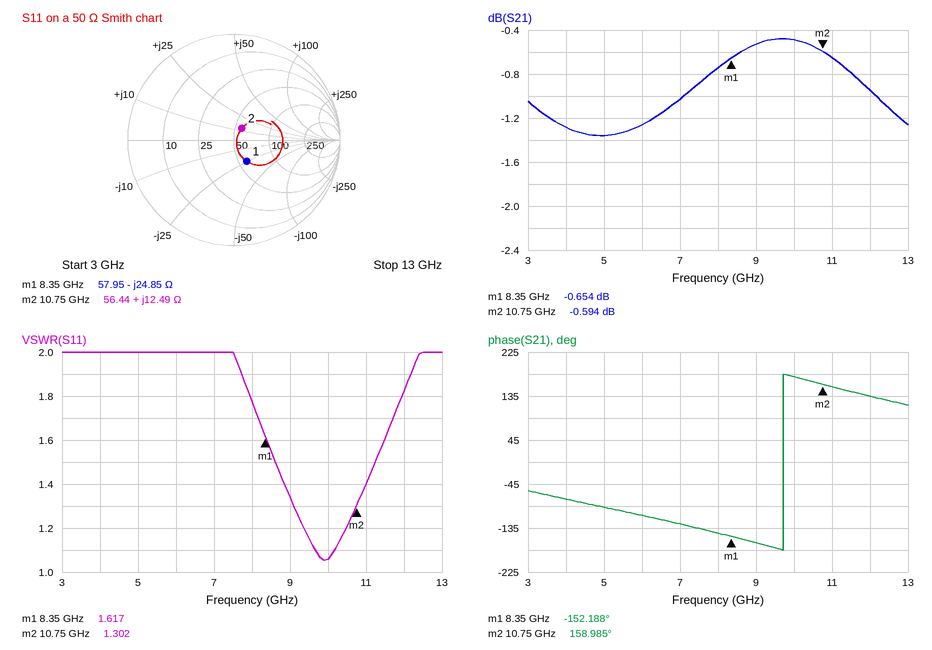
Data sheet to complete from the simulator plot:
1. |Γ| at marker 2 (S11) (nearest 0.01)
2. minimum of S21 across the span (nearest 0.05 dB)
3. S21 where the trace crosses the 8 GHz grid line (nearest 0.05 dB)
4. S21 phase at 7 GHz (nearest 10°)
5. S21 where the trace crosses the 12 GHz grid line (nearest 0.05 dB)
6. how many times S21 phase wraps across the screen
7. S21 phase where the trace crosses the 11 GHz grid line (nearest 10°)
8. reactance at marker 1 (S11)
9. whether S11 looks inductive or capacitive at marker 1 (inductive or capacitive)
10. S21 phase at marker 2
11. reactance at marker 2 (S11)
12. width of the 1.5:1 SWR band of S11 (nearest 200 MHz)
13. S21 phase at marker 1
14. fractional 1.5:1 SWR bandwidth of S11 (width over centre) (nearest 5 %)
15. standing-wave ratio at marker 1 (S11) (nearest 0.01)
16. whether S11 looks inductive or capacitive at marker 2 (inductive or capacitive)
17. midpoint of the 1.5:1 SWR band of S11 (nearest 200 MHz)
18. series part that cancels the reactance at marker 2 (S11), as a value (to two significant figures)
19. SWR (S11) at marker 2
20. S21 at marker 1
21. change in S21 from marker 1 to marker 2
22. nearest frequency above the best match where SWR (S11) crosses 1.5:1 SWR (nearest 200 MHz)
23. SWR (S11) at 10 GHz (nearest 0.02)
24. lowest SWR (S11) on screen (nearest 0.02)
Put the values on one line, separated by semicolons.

0.13; -1.35 dB; -0.75 dB; -130°; -0.95 dB; 1; 150°; -24.85 Ω; capacitive; 158.985°; +12.49 Ω; 2.6 GHz; -152.188°; 25 %; 1.62; inductive; 10.0 GHz; 1.2 pF; 1.302; -0.654 dB; 0.060 dB; 11.2 GHz; 1.06; 1.06
